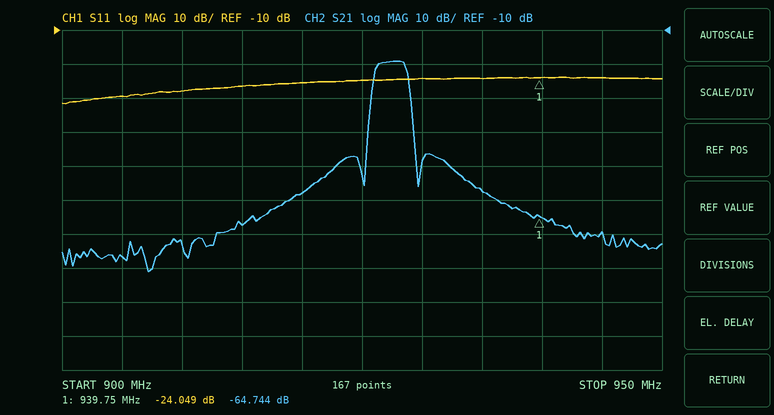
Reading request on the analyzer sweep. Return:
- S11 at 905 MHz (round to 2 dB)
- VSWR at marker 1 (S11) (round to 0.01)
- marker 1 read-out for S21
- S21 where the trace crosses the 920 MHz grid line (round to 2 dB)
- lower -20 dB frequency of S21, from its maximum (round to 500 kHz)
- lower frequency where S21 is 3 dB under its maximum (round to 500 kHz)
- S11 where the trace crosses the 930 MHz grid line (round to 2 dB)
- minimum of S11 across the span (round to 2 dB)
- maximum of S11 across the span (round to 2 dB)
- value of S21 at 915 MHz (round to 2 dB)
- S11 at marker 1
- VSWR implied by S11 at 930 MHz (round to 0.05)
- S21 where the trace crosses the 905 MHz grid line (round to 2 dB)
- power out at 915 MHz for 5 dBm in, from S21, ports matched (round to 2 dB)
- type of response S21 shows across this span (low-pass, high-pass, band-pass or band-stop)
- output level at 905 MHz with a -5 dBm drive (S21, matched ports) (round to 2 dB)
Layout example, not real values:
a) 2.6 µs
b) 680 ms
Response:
a) -30 dB
b) 1.13
c) -64.744 dB
d) -58 dB
e) 925.5 MHz
f) 926.0 MHz
g) -24 dB
h) -32 dB
i) -24 dB
j) -68 dB
k) -24.049 dB
l) 1.15
m) -76 dB
n) -62 dBm
o) band-pass
p) -82 dBm
